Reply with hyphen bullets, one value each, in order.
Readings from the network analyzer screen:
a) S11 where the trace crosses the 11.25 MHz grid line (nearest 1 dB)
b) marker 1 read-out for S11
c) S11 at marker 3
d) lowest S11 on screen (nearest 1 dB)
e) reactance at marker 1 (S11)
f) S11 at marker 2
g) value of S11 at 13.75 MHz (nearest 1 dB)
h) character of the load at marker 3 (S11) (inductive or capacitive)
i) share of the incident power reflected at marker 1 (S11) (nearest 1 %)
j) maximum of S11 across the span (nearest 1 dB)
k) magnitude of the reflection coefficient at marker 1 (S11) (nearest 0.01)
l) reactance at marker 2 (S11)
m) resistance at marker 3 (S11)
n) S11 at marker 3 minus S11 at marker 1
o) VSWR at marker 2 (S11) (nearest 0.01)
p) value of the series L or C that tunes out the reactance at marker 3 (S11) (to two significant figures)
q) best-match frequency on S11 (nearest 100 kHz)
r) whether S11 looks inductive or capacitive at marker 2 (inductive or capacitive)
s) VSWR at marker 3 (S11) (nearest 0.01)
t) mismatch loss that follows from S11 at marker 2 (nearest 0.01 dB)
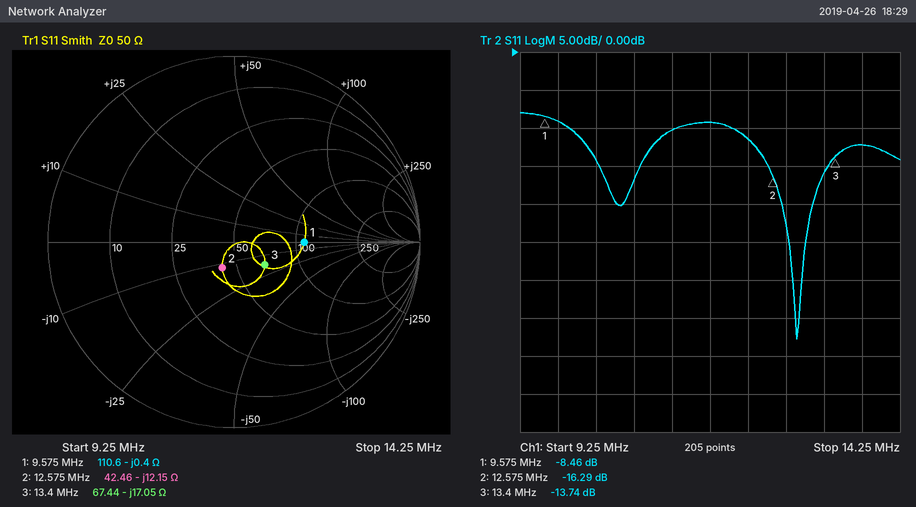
- -10 dB
- -8.46 dB
- -13.74 dB
- -38 dB
- -0.4 Ω
- -16.29 dB
- -12 dB
- capacitive
- 14 %
- -8 dB
- 0.38
- -12.15 Ω
- 67.44 Ω
- -5.28 dB
- 1.36
- 200 nH
- 12.9 MHz
- capacitive
- 1.52
- 0.10 dB
